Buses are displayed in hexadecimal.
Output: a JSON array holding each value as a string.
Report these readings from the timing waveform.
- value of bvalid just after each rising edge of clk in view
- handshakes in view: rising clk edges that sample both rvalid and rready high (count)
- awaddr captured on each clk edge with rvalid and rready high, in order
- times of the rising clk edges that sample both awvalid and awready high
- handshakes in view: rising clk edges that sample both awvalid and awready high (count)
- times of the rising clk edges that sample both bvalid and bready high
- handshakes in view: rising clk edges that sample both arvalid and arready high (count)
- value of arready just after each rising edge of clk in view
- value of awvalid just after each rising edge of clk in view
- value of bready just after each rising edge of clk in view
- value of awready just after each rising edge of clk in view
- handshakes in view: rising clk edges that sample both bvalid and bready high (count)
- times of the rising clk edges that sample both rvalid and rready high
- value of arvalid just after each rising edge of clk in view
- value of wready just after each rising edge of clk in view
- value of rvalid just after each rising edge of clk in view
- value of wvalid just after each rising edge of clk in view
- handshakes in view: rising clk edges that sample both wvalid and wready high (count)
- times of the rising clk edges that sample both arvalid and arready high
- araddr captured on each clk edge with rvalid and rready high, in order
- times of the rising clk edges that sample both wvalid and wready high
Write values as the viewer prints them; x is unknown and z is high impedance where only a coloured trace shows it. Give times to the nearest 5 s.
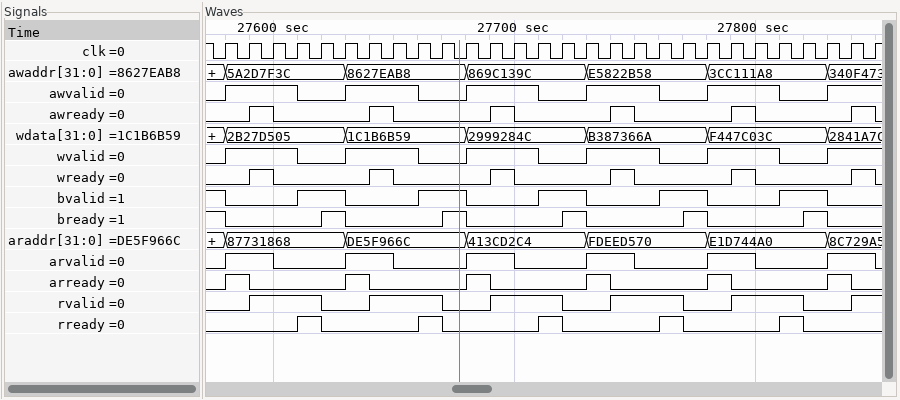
["0 0 0 1 1 0 0 0 1 1 0 0 0 1 1 0 0 0 1 1 0 0 0 1 1 0 0 0", "5", "5A2D7F3C, 8627EAB8, 869C139C, E5822B58, 3CC111A8", "27600 s, 27650 s, 27700 s, 27750 s, 27800 s, 27850 s", "6", "27580 s, 27630 s, 27680 s, 27730 s, 27780 s, 27830 s", "6", "1 0 0 0 0 1 0 0 0 0 1 0 0 0 0 1 0 0 0 0 1 0 0 0 0 1 0 0", "1 1 1 0 0 1 1 1 0 0 1 1 1 0 0 1 1 1 0 0 1 1 1 0 0 1 1 1", "0 0 0 0 1 0 0 0 0 1 0 0 0 0 1 0 0 0 0 1 0 0 0 0 1 0 0 0", "0 1 0 0 0 0 1 0 0 0 0 1 0 0 0 0 1 0 0 0 0 1 0 0 0 0 1 0", "6", "27620 s, 27670 s, 27720 s, 27770 s, 27820 s", "1 1 0 0 0 1 1 0 0 0 1 1 0 0 0 1 1 0 0 0 1 1 0 0 0 1 1 0", "0 1 0 0 0 0 1 0 0 0 0 1 0 0 0 0 1 0 0 0 0 1 0 0 0 0 1 0", "0 1 1 1 0 0 1 1 1 0 0 1 1 1 0 0 1 1 1 0 0 1 1 1 0 0 1 1", "1 1 1 0 0 1 1 1 0 0 1 1 1 0 0 1 1 1 0 0 1 1 1 0 0 1 1 1", "6", "27590 s, 27640 s, 27690 s, 27740 s, 27790 s, 27840 s", "87731868, DE5F966C, 413CD2C4, FDEED570, E1D744A0", "27600 s, 27650 s, 27700 s, 27750 s, 27800 s, 27850 s"]
